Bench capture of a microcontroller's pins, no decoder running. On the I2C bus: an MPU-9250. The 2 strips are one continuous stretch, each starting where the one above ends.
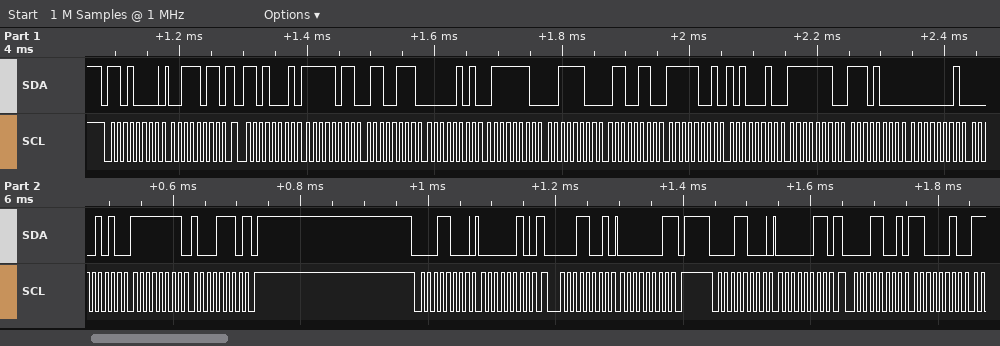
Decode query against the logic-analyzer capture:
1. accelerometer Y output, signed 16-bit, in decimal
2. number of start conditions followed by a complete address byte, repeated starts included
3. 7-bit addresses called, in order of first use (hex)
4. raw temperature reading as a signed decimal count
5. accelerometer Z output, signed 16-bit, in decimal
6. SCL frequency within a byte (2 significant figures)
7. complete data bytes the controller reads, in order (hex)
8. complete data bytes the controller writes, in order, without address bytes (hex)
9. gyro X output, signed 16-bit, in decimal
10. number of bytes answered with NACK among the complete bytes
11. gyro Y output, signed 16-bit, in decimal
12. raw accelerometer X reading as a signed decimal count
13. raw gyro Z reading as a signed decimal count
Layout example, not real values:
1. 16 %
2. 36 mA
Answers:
1. 1406
2. 6
3. 0x68 0x0C
4. -1630
5. 15462
6. 100 kHz
7. FB 67 05 7E 3C 66 F9 A2 FE E8 01 0A FF 8E 01 C2
8. 3B 02 03
9. -280
10. 2
11. 266
12. -1177
13. -114
